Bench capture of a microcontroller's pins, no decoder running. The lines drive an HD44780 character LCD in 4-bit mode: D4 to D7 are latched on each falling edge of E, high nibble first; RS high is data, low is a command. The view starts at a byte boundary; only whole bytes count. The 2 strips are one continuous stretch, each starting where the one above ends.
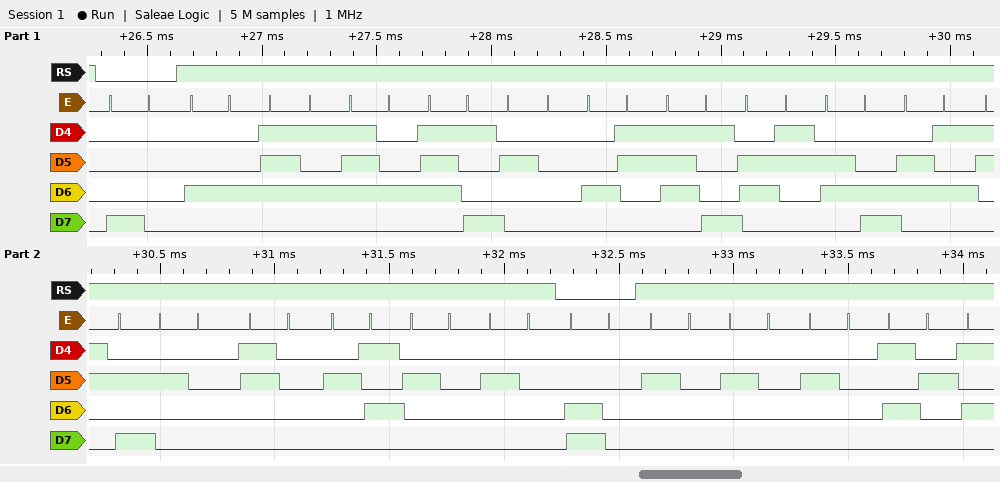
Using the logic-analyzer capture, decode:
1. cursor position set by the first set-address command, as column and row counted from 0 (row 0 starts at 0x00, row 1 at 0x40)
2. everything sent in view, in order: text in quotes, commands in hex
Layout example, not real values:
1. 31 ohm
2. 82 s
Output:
1. column 0, row 0
2. 0x80 "Duty Cycle: 0%  " 0xC0 "   R"
